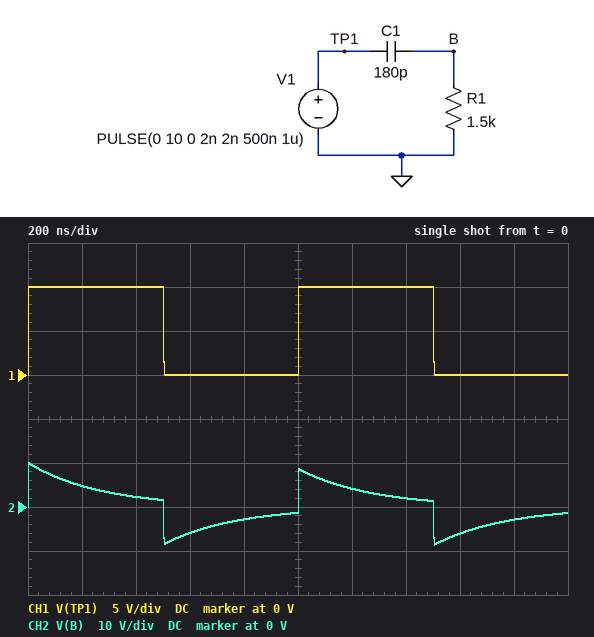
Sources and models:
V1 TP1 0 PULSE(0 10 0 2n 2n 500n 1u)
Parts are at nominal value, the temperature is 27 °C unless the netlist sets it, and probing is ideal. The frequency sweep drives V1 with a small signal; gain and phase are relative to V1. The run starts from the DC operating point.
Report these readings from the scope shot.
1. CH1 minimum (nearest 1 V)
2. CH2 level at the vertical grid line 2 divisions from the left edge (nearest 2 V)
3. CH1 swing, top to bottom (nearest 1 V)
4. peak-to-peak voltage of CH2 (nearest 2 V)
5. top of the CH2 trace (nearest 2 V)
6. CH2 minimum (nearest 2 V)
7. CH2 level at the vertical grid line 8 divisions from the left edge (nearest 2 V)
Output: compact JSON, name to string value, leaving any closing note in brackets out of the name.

{"CH1 minimum": "0 V", "CH2 level at the vertical grid line 2 divisions from the left edge": "2 V", "CH1 swing, top to bottom": "10 V", "peak-to-peak voltage of CH2": "18 V", "top of the CH2 trace": "10 V", "CH2 minimum": "-8 V", "CH2 level at the vertical grid line 8 divisions from the left edge": "-6 V"}
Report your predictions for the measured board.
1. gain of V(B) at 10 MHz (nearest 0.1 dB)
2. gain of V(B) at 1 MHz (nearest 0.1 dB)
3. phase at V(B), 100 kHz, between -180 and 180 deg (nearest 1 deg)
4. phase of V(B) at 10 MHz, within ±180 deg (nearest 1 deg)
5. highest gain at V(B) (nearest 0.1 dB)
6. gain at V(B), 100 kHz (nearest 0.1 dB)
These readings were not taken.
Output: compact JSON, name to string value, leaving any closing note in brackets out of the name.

{"gain of V(B) at 10 MHz": "0 dB", "gain of V(B) at 1 MHz": "-1.3 dB", "phase at V(B), 100 kHz, between -180 and 180 deg": "80 deg", "phase of V(B) at 10 MHz, within ±180 deg": "3 deg", "highest gain at V(B)": "0 dB", "gain at V(B), 100 kHz": "-15.5 dB"}
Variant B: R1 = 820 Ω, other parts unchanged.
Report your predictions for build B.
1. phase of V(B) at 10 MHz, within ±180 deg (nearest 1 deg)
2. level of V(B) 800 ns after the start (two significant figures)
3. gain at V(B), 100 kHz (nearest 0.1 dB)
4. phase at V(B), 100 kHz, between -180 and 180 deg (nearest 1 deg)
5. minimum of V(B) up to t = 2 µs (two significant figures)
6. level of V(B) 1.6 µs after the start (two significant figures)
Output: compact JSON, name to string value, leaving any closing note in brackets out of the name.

{"phase of V(B) at 10 MHz, within ±180 deg": "6 deg", "level of V(B) 800 ns after the start": "-1.3 V", "gain at V(B), 100 kHz": "-20.7 dB", "phase at V(B), 100 kHz, between -180 and 180 deg": "85 deg", "minimum of V(B) up to t = 2 µs": "-9.6 V", "level of V(B) 1.6 µs after the start": "-5.0 V"}
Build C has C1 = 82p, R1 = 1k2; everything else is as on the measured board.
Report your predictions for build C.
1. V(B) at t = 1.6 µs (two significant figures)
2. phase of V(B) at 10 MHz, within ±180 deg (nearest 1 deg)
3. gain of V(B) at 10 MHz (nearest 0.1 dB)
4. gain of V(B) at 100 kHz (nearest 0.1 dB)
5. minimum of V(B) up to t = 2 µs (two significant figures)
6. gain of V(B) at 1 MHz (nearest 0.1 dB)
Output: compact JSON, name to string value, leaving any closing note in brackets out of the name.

{"V(B) at t = 1.6 µs": "-3.7 V", "phase of V(B) at 10 MHz, within ±180 deg": "9 deg", "gain of V(B) at 10 MHz": "-0.1 dB", "gain of V(B) at 100 kHz": "-24.2 dB", "minimum of V(B) up to t = 2 µs": "-9.8 V", "gain of V(B) at 1 MHz": "-5.6 dB"}
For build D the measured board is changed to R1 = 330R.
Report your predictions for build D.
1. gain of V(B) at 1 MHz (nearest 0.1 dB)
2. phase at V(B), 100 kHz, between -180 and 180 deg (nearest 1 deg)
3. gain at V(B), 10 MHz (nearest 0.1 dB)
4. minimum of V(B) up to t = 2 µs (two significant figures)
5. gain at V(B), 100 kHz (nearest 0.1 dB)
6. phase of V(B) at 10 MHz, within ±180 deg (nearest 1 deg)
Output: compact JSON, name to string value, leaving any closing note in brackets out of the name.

{"gain of V(B) at 1 MHz": "-9.1 dB", "phase at V(B), 100 kHz, between -180 and 180 deg": "88 deg", "gain at V(B), 10 MHz": "-0.3 dB", "minimum of V(B) up to t = 2 µs": "-9.8 V", "gain at V(B), 100 kHz": "-28.6 dB", "phase of V(B) at 10 MHz, within ±180 deg": "15 deg"}
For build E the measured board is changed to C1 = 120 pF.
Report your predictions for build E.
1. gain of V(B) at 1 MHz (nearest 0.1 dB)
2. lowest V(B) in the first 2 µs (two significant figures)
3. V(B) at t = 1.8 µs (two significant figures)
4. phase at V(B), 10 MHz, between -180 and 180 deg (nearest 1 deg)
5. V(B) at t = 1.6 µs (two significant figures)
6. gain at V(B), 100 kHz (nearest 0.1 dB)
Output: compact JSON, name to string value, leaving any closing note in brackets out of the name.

{"gain of V(B) at 1 MHz": "-2.5 dB", "lowest V(B) in the first 2 µs": "-9.4 V", "V(B) at t = 1.8 µs": "-1.8 V", "phase at V(B), 10 MHz, between -180 and 180 deg": "5 deg", "V(B) at t = 1.6 µs": "-5.5 V", "gain at V(B), 100 kHz": "-19.0 dB"}
